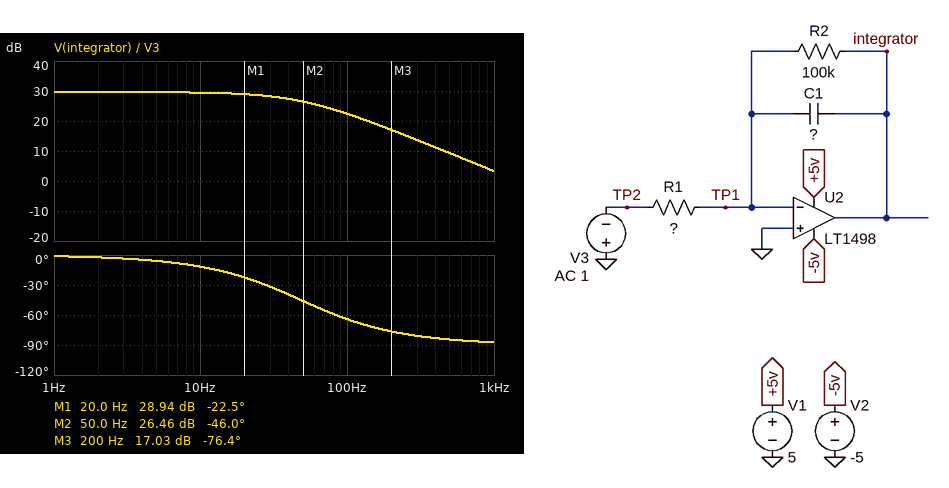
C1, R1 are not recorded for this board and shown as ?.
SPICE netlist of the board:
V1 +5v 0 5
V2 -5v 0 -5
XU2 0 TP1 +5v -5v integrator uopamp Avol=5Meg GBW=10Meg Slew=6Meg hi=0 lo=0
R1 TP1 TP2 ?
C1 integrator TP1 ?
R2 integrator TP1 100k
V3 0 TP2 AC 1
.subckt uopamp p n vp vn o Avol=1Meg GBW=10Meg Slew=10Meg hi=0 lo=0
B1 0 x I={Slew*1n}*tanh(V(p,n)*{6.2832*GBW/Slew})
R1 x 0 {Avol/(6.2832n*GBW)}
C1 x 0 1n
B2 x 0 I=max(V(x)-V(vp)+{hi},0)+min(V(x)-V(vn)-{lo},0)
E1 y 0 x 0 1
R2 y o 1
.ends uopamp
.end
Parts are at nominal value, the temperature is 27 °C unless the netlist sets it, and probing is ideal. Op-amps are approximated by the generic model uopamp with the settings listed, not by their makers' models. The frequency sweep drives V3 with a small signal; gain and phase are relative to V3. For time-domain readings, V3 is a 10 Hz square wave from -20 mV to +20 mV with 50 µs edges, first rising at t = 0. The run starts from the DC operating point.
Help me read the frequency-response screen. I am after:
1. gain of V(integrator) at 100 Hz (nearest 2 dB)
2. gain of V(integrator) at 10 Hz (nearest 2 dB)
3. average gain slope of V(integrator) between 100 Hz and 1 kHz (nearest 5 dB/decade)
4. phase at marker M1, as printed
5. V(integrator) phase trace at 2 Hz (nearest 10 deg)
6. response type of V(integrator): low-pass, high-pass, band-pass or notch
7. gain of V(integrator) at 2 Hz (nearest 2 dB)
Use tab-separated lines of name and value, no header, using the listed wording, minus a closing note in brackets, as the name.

gain of V(integrator) at 100 Hz	22 dB
gain of V(integrator) at 10 Hz	30 dB
average gain slope of V(integrator) between 100 Hz and 1 kHz	-20 dB/decade
phase at marker M1, as printed	-22.5 deg
V(integrator) phase trace at 2 Hz	0 deg
response type of V(integrator): low-pass, high-pass, band-pass or notch	low-pass
gain of V(integrator) at 2 Hz	30 dB
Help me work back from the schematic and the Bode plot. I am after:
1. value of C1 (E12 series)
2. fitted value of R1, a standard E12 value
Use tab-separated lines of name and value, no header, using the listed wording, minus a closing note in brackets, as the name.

value of C1	33 nF
fitted value of R1, a standard E12 value	3.3 kΩ
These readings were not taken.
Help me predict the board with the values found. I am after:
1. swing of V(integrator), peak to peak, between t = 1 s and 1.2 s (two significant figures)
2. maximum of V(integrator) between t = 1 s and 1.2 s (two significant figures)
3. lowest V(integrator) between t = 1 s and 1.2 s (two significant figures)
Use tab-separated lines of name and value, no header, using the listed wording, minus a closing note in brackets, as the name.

swing of V(integrator), peak to peak, between t = 1 s and 1.2 s	1.2 V
maximum of V(integrator) between t = 1 s and 1.2 s	610 mV
lowest V(integrator) between t = 1 s and 1.2 s	-610 mV
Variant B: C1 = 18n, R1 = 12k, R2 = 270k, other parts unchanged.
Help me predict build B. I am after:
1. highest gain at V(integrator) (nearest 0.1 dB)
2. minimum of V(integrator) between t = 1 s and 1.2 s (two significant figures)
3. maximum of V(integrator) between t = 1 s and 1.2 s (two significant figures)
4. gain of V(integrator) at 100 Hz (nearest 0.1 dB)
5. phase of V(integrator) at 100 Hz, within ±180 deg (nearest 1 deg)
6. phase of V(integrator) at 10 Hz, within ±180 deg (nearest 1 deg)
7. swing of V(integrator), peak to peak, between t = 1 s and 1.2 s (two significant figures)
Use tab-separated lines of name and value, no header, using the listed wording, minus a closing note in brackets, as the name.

highest gain at V(integrator)	27.0 dB
minimum of V(integrator) between t = 1 s and 1.2 s	-450 mV
maximum of V(integrator) between t = 1 s and 1.2 s	450 mV
gain of V(integrator) at 100 Hz	16.9 dB
phase of V(integrator) at 100 Hz, within ±180 deg	-72 deg
phase of V(integrator) at 10 Hz, within ±180 deg	-17 deg
swing of V(integrator), peak to peak, between t = 1 s and 1.2 s	900 mV
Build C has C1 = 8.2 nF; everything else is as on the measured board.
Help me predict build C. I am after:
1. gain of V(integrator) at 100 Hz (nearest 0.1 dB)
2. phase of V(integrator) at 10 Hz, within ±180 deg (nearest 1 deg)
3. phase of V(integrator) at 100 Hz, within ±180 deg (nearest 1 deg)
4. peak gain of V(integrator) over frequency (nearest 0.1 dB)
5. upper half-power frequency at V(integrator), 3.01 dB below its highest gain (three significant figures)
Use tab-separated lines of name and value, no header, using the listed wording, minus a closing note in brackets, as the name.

gain of V(integrator) at 100 Hz	28.6 dB
phase of V(integrator) at 10 Hz, within ±180 deg	-3 deg
phase of V(integrator) at 100 Hz, within ±180 deg	-27 deg
peak gain of V(integrator) over frequency	29.6 dB
upper half-power frequency at V(integrator), 3.01 dB below its highest gain	194 Hz
